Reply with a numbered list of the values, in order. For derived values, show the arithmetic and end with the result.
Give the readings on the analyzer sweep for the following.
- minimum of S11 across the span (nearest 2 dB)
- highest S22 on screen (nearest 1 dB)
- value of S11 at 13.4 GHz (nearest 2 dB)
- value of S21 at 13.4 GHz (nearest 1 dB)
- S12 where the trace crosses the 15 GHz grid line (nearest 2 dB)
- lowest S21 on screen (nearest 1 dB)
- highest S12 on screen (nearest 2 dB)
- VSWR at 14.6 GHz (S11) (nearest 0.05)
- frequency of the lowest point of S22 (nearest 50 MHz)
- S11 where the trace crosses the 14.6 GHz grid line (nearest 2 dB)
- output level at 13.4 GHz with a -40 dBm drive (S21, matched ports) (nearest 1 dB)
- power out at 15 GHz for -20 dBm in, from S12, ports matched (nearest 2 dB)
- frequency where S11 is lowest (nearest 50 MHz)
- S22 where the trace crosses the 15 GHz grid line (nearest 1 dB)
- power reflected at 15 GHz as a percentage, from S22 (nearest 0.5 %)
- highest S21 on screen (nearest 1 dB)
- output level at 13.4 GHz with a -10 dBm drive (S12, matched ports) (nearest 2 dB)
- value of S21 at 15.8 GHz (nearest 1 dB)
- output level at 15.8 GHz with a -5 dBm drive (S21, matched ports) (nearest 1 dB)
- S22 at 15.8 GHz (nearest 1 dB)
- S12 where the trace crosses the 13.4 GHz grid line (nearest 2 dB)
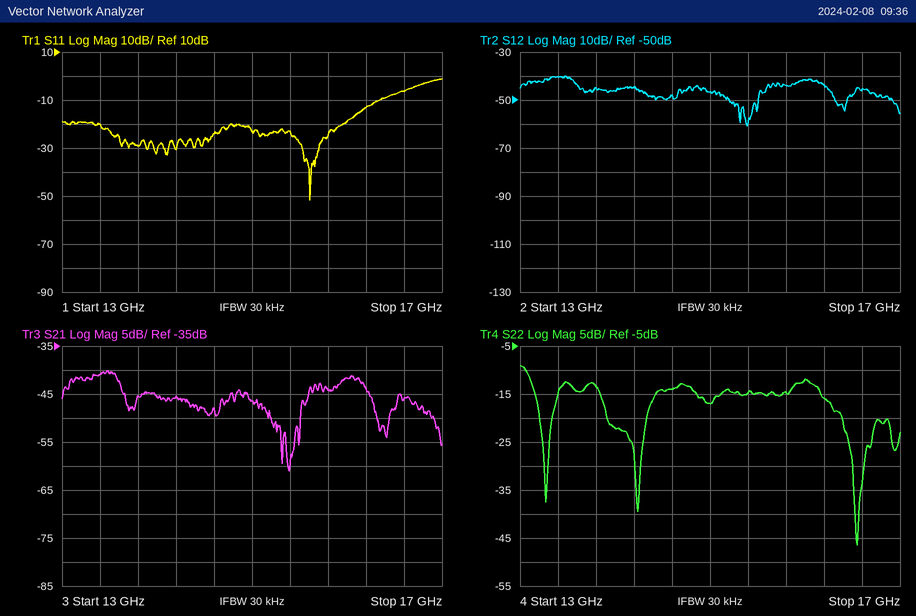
1. -52 dB
2. -9 dB
3. -20 dB
4. -41 dB
5. -46 dB
6. -61 dB
7. -40 dB
8. |Γ| = 10^(-24/20) = 0.0631; VSWR = (1 + 0.0631)/(1 − 0.0631) ≈ 1.13, so 1.15 to the nearest 0.05
9. 16.55 GHz
10. -24 dB
11. -40 dBm + (-41 dB) = -81 dBm
12. -20 dBm + (-46 dB) = -66 dBm
13. 15.60 GHz
14. -17 dB
15. 10^(-17/10) ≈ 2.0 %
16. -40 dB
17. -10 dBm + (-40 dB) = -50 dBm
18. -44 dB
19. -5 dBm + (-44 dB) = -49 dBm
20. -15 dB
21. -40 dB
